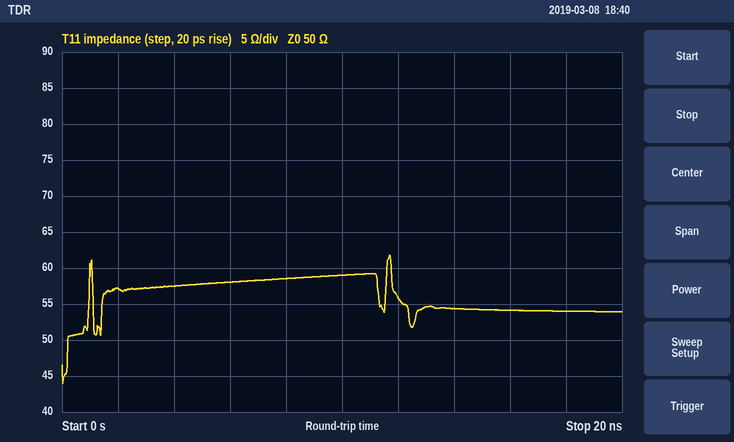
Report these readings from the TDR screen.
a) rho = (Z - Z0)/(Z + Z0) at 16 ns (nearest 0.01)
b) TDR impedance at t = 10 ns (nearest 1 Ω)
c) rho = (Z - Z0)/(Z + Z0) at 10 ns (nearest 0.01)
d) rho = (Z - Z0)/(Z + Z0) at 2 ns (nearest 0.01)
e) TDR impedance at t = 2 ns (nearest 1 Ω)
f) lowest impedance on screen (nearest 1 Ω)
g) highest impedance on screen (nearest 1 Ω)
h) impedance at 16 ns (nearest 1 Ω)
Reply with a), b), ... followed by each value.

a) +0.04
b) 59 Ω
c) +0.08
d) +0.07
e) 57 Ω
f) 44 Ω
g) 62 Ω
h) 54 Ω
